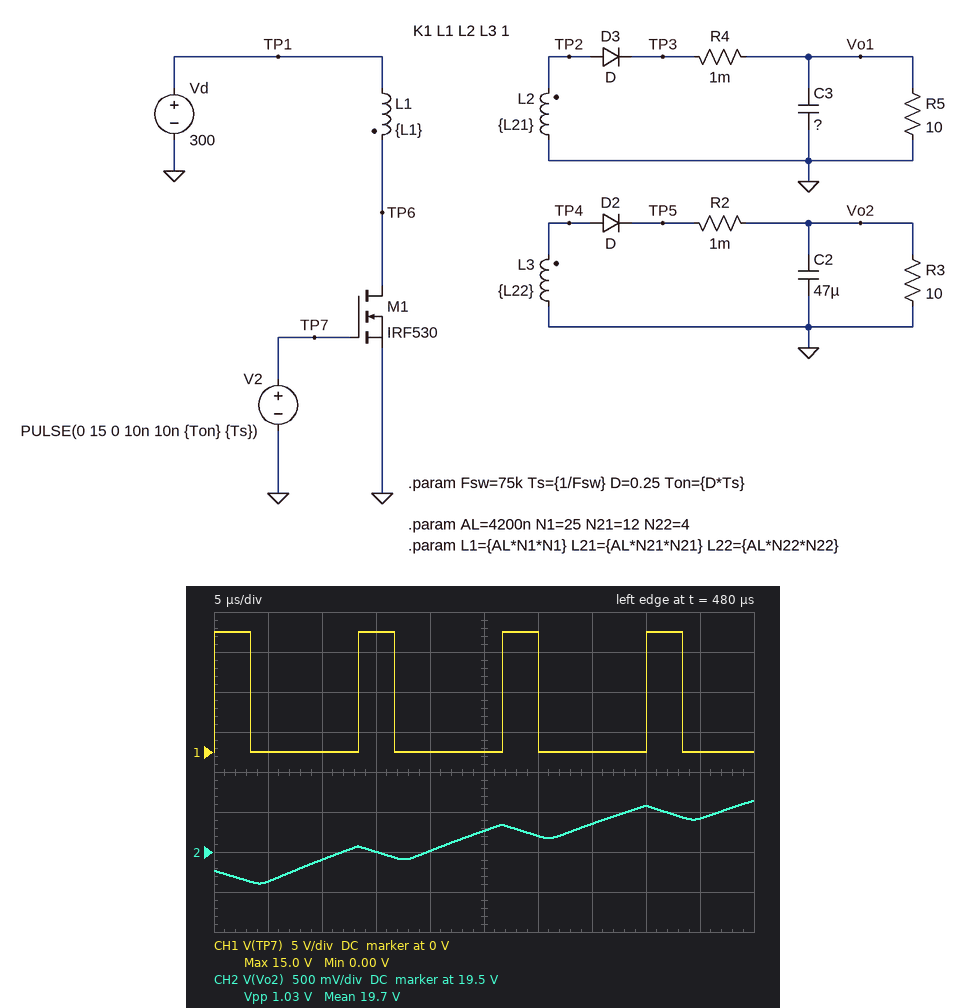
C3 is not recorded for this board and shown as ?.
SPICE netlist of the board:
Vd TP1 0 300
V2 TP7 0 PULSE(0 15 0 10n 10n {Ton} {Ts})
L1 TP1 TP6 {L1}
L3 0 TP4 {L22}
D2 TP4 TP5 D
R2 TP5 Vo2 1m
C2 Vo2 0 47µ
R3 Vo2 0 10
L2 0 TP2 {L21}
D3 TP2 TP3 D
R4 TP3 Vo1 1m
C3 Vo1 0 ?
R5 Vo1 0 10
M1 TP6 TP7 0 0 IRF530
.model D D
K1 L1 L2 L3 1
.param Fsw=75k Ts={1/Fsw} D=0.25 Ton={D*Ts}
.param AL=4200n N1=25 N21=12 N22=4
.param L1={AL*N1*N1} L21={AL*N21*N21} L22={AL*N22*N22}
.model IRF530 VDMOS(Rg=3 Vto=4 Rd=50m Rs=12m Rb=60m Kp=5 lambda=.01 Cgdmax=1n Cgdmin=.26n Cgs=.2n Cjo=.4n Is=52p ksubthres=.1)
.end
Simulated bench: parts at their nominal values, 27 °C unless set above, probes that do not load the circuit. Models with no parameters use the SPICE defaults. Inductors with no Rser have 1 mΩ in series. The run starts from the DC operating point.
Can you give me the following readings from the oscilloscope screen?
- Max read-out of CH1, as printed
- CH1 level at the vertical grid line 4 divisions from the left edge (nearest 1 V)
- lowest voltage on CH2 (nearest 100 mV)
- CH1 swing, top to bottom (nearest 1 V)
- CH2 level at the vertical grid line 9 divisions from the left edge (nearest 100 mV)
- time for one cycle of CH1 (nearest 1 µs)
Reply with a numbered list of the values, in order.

1. 15.0 V
2. 0 V
3. 19.1 V
4. 15 V
5. 19.9 V
6. 13 µs
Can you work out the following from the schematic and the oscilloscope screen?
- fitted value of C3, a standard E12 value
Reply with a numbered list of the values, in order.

1. 27 µF
